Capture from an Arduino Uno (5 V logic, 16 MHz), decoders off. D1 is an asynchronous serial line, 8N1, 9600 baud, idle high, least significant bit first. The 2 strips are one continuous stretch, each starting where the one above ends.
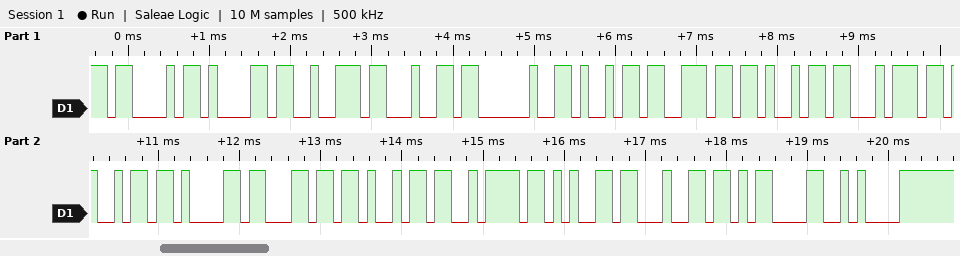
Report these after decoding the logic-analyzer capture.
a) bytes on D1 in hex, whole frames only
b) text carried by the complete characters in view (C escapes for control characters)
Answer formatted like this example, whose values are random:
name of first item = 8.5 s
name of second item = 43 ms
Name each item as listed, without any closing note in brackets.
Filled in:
bytes on D1 in hex, whole frames only = 43 61 72 64 20 69 6E 69 74 69 61 6C 69 7A 65 64 0D 0A
text carried by the complete characters in view = "Card initialized\r\n"
